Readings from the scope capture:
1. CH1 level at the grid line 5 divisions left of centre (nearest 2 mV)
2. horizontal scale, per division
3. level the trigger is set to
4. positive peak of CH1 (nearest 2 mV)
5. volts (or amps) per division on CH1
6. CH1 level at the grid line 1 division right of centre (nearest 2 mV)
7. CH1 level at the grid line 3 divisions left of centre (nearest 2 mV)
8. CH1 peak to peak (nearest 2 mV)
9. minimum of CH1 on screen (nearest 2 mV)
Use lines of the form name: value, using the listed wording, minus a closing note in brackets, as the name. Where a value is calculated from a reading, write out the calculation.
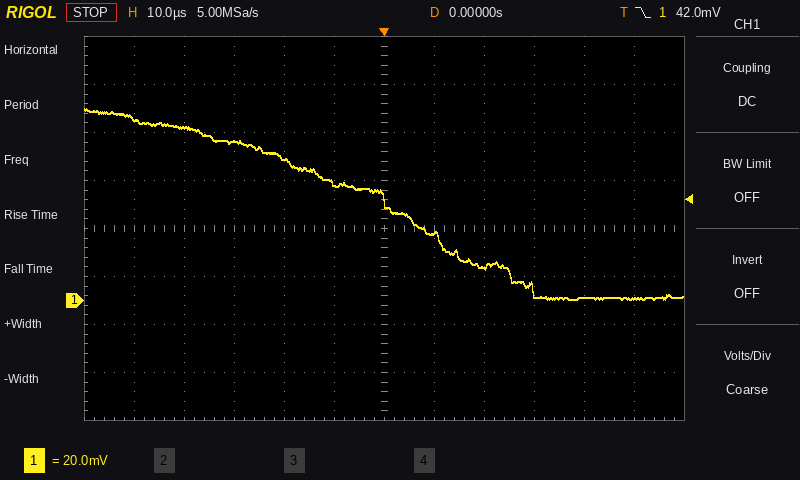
CH1 level at the grid line 5 divisions left of centre: 76 mV
horizontal scale, per division: 10 µs
level the trigger is set to: 42.0 mV
positive peak of CH1: 80 mV
volts (or amps) per division on CH1: 20 mV
CH1 level at the grid line 1 division right of centre: 28 mV
CH1 level at the grid line 3 divisions left of centre: 66 mV
CH1 peak to peak: 80 mV − (0 mV) = 80 mV
minimum of CH1 on screen: 0 mV
